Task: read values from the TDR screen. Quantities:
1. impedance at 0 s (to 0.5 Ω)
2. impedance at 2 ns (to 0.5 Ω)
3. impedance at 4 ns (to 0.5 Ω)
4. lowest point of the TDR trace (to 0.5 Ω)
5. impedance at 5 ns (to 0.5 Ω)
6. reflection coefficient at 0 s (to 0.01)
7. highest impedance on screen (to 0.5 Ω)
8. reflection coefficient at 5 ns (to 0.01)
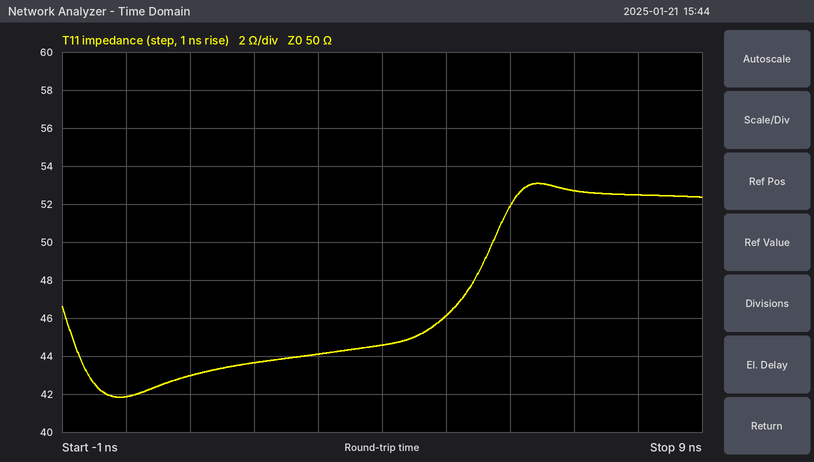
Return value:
42.0 Ω
43.5 Ω
44.5 Ω
42.0 Ω
46.0 Ω
-0.09
53.0 Ω
-0.04
